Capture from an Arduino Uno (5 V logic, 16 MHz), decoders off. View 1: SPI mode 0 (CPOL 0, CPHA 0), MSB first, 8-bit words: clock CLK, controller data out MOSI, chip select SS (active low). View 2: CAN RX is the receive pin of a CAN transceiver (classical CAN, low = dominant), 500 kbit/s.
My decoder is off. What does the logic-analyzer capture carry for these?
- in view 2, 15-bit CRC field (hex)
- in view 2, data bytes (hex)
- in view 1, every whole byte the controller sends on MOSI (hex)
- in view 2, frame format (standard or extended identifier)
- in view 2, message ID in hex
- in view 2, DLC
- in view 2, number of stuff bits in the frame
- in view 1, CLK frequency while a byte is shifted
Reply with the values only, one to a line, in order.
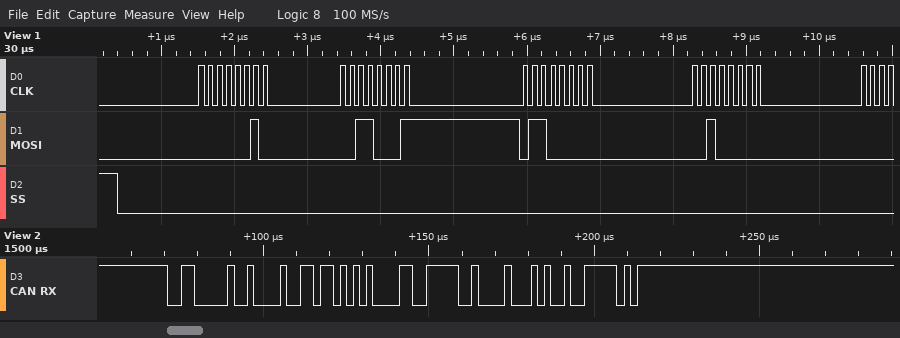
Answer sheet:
0x149F
DA A1 9F 42
02 31 60 20
standard
0x301
4
3
8 MHz
